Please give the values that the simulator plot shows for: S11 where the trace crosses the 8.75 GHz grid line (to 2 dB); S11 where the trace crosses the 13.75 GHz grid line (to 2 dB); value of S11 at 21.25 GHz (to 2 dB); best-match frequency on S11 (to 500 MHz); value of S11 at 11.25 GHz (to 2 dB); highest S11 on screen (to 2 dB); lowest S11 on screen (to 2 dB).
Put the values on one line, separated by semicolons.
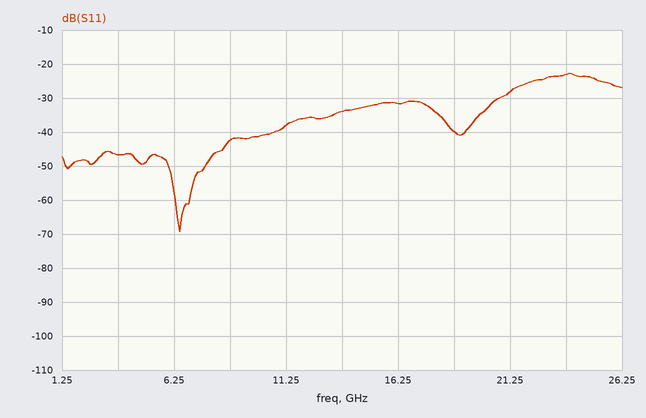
-42 dB; -34 dB; -28 dB; 6.5 GHz; -38 dB; -22 dB; -70 dB
